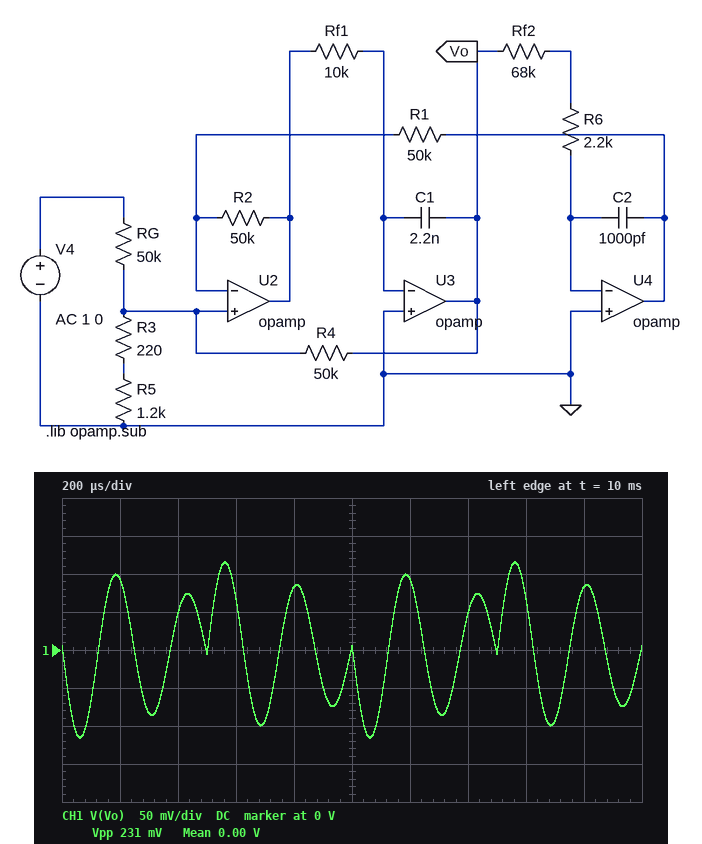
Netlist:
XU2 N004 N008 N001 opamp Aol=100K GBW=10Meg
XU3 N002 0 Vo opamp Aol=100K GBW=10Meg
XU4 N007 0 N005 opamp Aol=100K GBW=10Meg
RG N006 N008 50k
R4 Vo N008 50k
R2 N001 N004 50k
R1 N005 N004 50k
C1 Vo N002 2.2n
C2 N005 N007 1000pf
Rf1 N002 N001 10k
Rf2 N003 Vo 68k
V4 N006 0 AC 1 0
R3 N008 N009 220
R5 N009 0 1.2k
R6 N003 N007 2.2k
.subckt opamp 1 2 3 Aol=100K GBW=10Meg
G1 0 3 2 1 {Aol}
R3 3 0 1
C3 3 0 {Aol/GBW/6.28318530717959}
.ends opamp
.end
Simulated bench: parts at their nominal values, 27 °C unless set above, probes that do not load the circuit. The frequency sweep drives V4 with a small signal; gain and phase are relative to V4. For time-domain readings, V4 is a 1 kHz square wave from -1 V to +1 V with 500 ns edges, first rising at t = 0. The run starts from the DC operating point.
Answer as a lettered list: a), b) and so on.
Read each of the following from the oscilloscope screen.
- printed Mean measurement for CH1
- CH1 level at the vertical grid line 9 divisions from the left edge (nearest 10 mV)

a) 0.00 V
b) 80 mV
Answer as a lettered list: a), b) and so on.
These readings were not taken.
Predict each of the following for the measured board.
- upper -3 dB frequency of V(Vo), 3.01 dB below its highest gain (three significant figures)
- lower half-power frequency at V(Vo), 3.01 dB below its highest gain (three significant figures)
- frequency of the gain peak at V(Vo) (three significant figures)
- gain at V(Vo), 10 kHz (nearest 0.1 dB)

a) 4.24 kHz
b) 3.86 kHz
c) 4.05 kHz
d) -26.7 dB
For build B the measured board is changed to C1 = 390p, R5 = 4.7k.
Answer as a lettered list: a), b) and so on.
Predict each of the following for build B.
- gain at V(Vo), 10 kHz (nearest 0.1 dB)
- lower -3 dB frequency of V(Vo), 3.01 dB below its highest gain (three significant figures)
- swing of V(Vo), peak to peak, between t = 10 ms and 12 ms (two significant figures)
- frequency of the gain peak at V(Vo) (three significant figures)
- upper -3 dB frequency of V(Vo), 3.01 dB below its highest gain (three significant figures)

a) 0 dB
b) 6.84 kHz
c) 1.8 V
d) 9.61 kHz
e) 13.5 kHz
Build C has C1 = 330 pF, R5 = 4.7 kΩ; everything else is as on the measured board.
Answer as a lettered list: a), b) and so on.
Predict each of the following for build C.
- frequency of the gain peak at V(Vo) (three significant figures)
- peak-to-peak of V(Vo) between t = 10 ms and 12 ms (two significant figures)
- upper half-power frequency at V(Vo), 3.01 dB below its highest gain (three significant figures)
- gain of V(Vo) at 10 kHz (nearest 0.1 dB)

a) 10.4 kHz
b) 1.9 V
c) 15.1 kHz
d) 0 dB
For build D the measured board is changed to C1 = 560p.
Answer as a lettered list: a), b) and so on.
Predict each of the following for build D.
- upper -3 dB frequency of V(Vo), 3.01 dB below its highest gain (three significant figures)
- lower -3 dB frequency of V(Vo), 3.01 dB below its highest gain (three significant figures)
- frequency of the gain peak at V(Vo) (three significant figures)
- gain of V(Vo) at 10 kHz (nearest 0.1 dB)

a) 8.80 kHz
b) 7.30 kHz
c) 8.02 kHz
d) -8.1 dB
